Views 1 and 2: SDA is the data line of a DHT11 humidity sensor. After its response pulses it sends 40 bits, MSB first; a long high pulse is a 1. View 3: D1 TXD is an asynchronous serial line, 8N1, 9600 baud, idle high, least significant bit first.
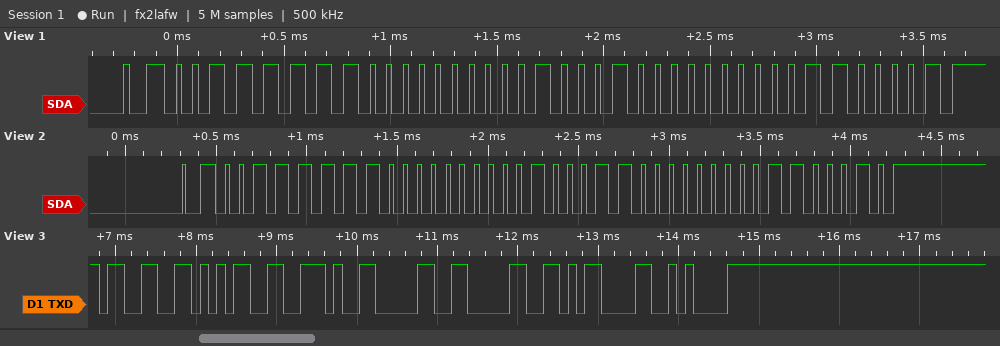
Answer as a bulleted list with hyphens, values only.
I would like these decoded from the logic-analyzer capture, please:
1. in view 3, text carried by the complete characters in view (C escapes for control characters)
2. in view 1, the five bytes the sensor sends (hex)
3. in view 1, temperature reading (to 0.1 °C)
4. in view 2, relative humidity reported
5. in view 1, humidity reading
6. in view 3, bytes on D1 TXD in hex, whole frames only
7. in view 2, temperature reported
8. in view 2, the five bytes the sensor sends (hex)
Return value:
- "35.00\r\n"
- 3F 00 22 00 61
- 34.0 °C
- 63 %
- 63 %
- 33 35 2E 30 30 0D 0A
- 35.0 °C
- 3F 00 23 00 62
